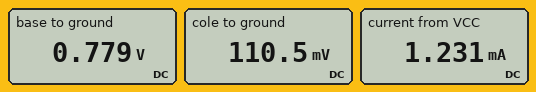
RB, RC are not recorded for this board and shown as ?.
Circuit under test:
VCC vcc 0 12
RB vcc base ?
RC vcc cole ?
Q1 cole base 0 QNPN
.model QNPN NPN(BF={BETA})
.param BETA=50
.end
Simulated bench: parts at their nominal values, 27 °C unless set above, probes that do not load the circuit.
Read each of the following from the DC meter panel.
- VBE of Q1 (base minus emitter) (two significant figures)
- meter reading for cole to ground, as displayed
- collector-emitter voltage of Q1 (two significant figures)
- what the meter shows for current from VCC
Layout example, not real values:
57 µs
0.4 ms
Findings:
780 mV
110.5 mV
110 mV
1.231 mA
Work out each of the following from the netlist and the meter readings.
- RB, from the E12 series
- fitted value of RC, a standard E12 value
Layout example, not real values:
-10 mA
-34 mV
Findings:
270 kΩ
10 kΩ
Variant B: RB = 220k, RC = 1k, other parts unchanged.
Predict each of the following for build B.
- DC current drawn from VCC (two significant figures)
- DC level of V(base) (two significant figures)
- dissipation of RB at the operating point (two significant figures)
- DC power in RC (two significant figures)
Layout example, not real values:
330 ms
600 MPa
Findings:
2.6 mA
800 mV
570 µW
6.5 mW
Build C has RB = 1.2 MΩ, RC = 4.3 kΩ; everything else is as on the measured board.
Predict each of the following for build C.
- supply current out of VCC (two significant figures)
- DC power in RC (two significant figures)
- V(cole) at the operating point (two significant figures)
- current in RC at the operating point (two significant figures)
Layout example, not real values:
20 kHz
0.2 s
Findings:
480 µA
940 µW
10 V
470 µA
